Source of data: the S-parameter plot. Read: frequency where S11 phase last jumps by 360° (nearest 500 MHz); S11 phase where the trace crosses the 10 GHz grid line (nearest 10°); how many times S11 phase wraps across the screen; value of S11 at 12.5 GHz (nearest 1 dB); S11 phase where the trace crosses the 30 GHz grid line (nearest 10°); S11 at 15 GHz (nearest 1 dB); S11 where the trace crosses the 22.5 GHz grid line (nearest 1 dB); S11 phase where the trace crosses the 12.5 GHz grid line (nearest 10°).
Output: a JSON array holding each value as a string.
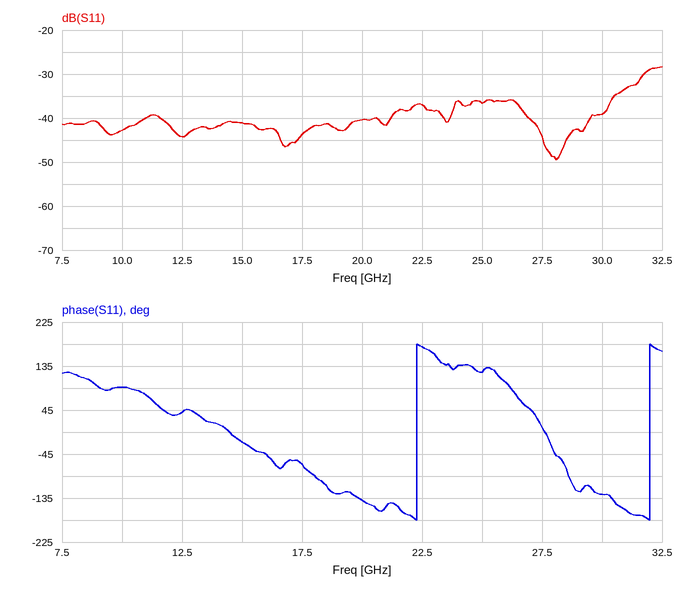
["32.0 GHz", "90°", "2", "-44 dB", "-130°", "-41 dB", "-37 dB", "40°"]
